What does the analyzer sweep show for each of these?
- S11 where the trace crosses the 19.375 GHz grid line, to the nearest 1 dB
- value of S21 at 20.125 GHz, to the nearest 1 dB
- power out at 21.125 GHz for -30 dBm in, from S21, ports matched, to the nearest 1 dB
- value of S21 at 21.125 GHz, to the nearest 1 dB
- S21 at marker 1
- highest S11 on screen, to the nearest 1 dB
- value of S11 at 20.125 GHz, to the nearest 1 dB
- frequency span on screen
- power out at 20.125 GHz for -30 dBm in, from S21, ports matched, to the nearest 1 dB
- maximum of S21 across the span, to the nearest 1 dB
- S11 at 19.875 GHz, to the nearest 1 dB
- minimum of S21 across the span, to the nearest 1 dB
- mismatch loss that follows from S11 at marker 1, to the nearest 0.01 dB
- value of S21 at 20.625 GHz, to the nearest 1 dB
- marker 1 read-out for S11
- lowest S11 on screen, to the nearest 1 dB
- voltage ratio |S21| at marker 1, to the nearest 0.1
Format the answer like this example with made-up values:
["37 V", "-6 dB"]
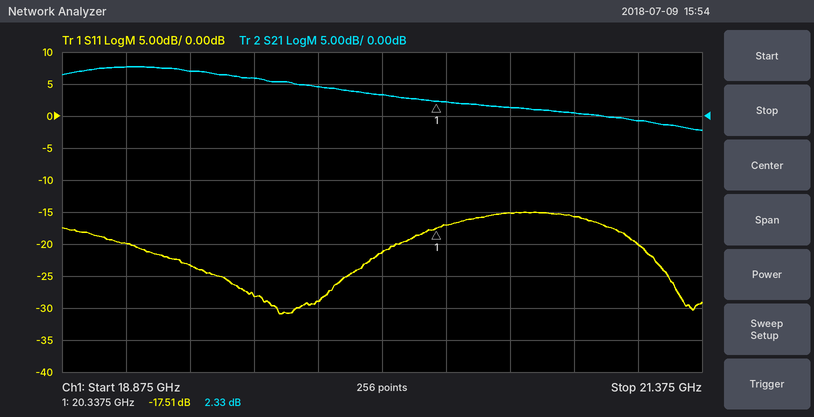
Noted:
["-23 dB", "3 dB", "-31 dBm", "-1 dB", "2.33 dB", "-15 dB", "-21 dB", "2.5 GHz", "-27 dBm", "8 dB", "-29 dB", "-2 dB", "0.08 dB", "1 dB", "-17.51 dB", "-31 dB", "1.3"]
